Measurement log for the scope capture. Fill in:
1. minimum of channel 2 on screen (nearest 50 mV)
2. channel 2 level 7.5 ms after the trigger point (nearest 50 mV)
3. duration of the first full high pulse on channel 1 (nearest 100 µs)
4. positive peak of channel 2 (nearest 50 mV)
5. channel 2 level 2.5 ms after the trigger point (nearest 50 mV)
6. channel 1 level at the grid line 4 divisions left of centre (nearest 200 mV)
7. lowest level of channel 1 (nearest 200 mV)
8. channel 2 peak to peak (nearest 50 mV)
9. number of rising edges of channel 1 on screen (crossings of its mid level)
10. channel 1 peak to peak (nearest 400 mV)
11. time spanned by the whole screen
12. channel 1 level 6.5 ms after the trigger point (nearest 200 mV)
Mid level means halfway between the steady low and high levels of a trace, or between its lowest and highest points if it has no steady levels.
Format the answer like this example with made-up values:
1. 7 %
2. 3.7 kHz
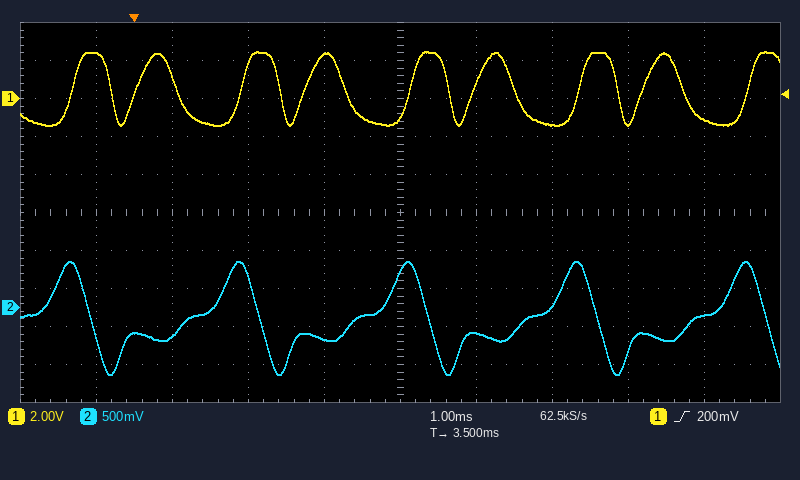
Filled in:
1. -900 mV
2. -100 mV
3. 500 µs
4. 600 mV
5. -400 mV
6. 2.4 V
7. -1.4 V
8. 1.50 V
9. 9
10. 4.0 V
11. 10 ms
12. -1.2 V
